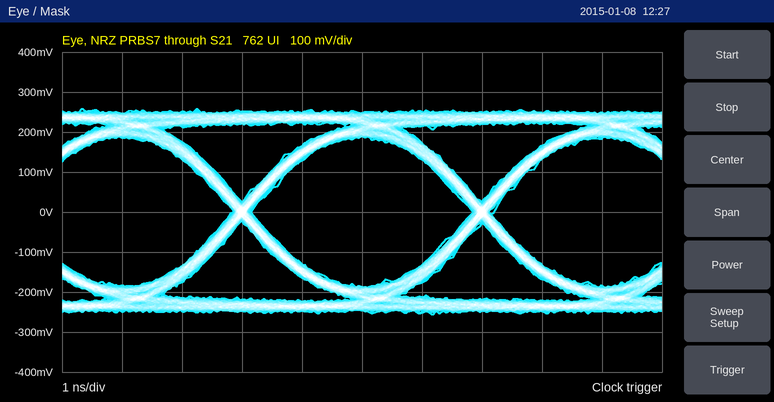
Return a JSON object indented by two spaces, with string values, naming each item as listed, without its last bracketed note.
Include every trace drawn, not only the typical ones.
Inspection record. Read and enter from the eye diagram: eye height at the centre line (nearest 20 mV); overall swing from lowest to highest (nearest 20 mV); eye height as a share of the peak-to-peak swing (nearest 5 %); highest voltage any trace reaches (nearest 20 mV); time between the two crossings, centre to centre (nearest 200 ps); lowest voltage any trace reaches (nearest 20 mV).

{
  "eye height at the centre line": "380 mV",
  "overall swing from lowest to highest": "520 mV",
  "eye height as a share of the peak-to-peak swing": "75 %",
  "highest voltage any trace reaches": "260 mV",
  "time between the two crossings, centre to centre": "4.0 ns",
  "lowest voltage any trace reaches": "-260 mV"
}
